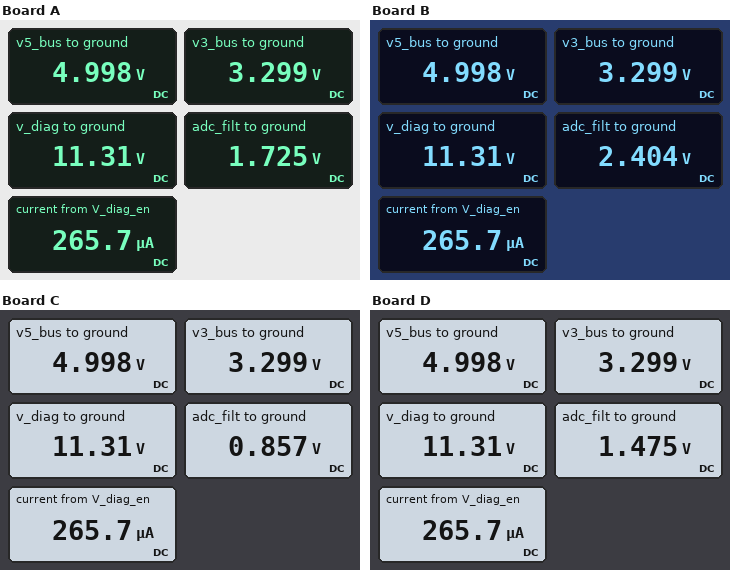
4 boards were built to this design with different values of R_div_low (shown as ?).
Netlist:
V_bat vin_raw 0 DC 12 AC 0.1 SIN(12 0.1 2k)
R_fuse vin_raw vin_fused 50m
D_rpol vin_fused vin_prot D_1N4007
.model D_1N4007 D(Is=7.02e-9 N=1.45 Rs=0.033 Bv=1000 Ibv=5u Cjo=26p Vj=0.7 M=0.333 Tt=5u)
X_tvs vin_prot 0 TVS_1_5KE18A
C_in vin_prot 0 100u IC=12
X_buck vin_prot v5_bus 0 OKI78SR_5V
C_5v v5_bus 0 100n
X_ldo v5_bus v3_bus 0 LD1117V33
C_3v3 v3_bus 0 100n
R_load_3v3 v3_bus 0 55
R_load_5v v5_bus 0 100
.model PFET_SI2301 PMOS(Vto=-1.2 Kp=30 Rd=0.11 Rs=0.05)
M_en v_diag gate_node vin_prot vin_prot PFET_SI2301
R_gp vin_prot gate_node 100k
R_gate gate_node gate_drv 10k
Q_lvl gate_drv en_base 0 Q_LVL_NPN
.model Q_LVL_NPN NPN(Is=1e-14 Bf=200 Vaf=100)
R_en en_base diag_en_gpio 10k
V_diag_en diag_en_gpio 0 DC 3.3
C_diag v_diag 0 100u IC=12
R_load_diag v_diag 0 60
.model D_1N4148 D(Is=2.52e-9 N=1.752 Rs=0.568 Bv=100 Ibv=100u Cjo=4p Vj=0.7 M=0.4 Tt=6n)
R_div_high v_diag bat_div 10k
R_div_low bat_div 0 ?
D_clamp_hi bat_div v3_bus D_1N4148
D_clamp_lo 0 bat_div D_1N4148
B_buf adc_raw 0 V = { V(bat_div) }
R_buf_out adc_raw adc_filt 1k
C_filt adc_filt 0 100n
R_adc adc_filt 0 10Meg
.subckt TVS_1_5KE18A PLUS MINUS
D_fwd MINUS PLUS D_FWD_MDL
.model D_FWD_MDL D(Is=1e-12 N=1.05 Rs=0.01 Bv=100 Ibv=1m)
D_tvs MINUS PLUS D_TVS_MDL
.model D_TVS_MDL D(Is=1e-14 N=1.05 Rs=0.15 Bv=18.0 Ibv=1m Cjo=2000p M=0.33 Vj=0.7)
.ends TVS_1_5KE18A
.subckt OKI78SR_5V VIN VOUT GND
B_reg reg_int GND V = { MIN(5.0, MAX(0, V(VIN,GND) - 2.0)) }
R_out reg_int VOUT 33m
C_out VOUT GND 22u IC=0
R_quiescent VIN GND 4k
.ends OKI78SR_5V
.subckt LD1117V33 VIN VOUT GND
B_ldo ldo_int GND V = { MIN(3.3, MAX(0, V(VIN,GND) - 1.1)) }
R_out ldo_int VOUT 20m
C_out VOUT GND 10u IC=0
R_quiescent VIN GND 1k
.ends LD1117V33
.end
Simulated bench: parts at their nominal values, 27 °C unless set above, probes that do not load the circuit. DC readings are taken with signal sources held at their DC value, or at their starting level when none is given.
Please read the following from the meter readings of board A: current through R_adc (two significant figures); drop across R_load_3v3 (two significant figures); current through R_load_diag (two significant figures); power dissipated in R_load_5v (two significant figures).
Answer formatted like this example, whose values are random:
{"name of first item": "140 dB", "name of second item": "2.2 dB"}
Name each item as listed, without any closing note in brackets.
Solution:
{"current through R_adc": "170 nA", "drop across R_load_3v3": "3.3 V", "current through R_load_diag": "190 mA", "power dissipated in R_load_5v": "250 mW"}
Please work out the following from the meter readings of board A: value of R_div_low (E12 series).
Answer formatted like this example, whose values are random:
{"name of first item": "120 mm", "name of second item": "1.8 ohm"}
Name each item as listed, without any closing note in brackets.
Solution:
{"value of R_div_low": "1.8 kΩ"}
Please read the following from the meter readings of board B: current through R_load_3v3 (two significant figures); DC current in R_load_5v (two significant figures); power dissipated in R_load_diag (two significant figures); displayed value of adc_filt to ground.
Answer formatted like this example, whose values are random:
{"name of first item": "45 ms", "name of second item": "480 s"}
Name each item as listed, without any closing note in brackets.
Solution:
{"current through R_load_3v3": "60 mA", "DC current in R_load_5v": "50 mA", "power dissipated in R_load_diag": "2.1 W", "displayed value of adc_filt to ground": "2.404 V"}
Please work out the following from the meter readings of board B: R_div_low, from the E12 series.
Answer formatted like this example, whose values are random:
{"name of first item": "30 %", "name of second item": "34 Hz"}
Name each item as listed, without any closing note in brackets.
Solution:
{"R_div_low, from the E12 series": "2.7 kΩ"}
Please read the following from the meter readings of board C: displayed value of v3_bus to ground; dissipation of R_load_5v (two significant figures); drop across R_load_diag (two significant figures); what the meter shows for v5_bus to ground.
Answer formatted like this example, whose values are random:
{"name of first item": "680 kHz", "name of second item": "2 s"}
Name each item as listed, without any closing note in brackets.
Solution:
{"displayed value of v3_bus to ground": "3.299 V", "dissipation of R_load_5v": "250 mW", "drop across R_load_diag": "11 V", "what the meter shows for v5_bus to ground": "4.998 V"}
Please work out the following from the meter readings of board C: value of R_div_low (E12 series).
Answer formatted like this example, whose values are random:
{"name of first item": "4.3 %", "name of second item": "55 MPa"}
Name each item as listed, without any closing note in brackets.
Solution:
{"value of R_div_low": "820 Ω"}
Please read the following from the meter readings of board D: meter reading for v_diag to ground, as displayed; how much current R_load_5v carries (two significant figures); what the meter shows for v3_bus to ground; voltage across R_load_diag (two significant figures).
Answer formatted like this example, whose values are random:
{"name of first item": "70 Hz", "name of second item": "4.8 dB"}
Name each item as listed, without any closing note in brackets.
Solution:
{"meter reading for v_diag to ground, as displayed": "11.31 V", "how much current R_load_5v carries": "50 mA", "what the meter shows for v3_bus to ground": "3.299 V", "voltage across R_load_diag": "11 V"}
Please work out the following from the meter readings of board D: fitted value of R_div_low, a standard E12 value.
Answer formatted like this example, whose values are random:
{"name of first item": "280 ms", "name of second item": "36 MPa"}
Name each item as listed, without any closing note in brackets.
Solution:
{"fitted value of R_div_low, a standard E12 value": "1.5 kΩ"}
